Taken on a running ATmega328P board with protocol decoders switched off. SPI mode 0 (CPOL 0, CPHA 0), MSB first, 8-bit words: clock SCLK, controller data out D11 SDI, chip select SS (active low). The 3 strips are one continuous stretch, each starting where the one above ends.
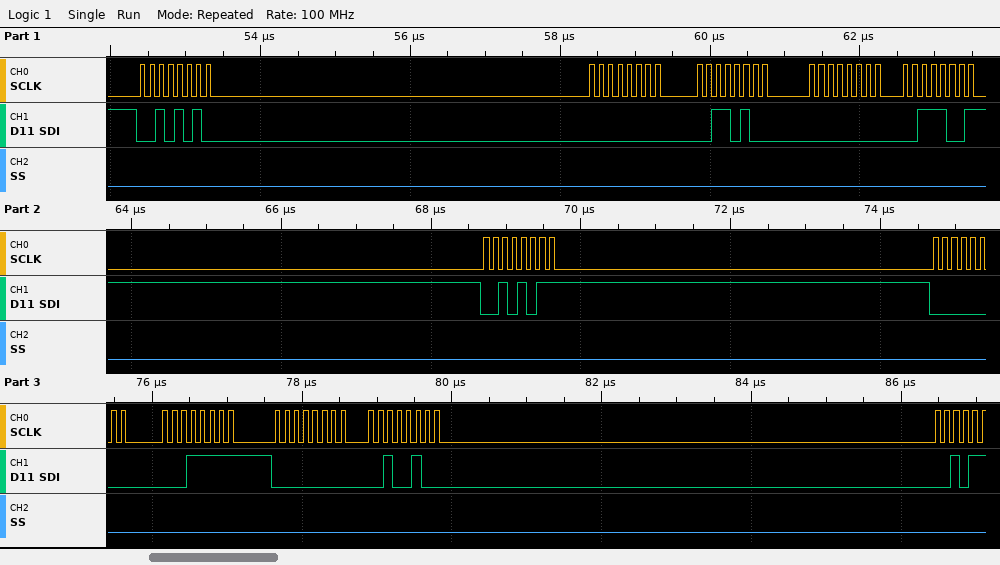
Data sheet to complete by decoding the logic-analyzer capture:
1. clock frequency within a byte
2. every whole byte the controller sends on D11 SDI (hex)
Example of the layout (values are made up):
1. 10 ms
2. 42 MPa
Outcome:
1. 8 MHz
2. 0x2A 0x00 0x34 0x00 0x39 0x2B 0x00 0x1F 0x00 0x24
